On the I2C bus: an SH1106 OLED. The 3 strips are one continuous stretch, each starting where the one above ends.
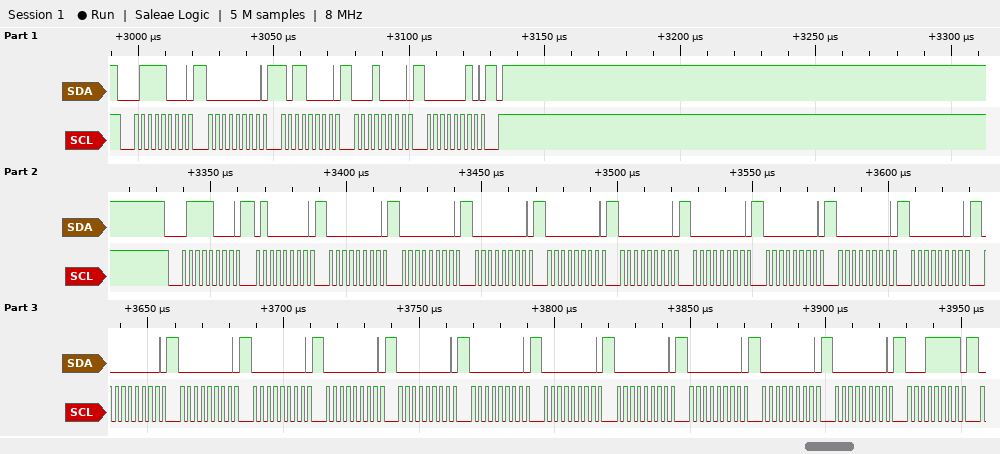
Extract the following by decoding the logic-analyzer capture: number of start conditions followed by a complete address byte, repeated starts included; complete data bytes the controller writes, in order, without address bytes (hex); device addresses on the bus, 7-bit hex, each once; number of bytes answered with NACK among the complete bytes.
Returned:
2
00 B0 10 02 40 00 00 00 00 00 00 00 00 00 00 00 00 00 00 00 00 00 00 00 00 1F
0x3C
0
